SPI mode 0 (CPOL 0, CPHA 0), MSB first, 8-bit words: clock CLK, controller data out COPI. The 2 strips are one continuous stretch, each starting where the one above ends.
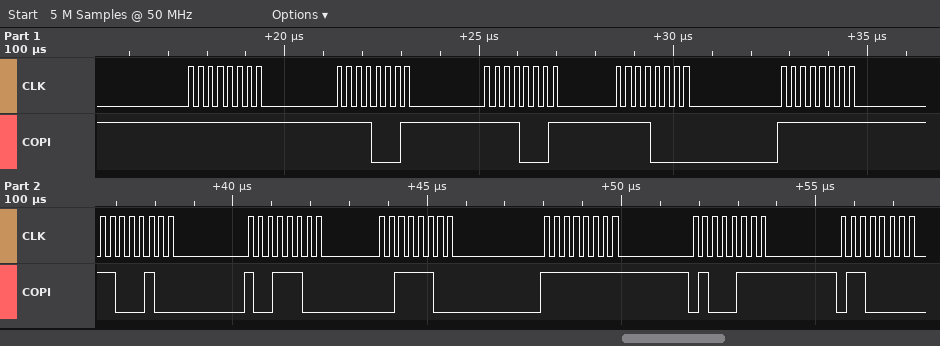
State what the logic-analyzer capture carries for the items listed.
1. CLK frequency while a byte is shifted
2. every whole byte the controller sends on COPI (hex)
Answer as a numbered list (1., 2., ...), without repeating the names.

1. 4 MHz
2. FF F1 F1 F0 FF C4 9C 3C FF 47 60
